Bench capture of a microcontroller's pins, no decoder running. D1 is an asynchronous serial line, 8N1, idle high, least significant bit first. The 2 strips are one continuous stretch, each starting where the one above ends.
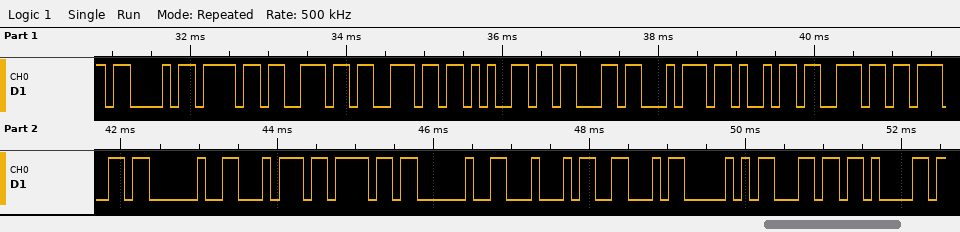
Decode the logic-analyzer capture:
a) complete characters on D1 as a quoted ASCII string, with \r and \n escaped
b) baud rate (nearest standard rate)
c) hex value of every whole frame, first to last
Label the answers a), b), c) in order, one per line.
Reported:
a) "Connecting to DFPla"
b) 9600 baud
c) 43 6F 6E 6E 65 63 74 69 6E 67 20 74 6F 20 44 46 50 6C 61
